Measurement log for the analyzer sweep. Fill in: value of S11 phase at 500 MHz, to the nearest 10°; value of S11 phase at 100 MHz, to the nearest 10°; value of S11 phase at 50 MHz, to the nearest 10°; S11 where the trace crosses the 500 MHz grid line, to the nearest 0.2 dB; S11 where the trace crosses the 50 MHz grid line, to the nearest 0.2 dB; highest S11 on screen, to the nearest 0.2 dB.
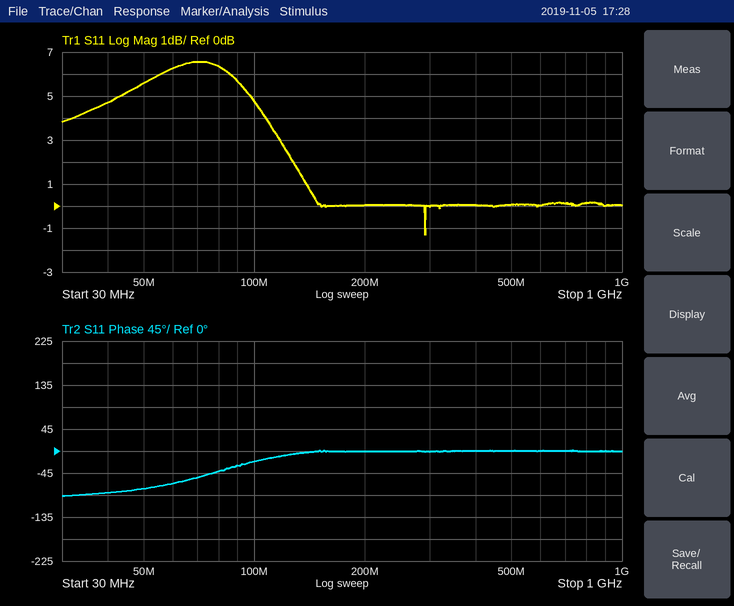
0°
-20°
-80°
0.0 dB
5.6 dB
6.6 dB
